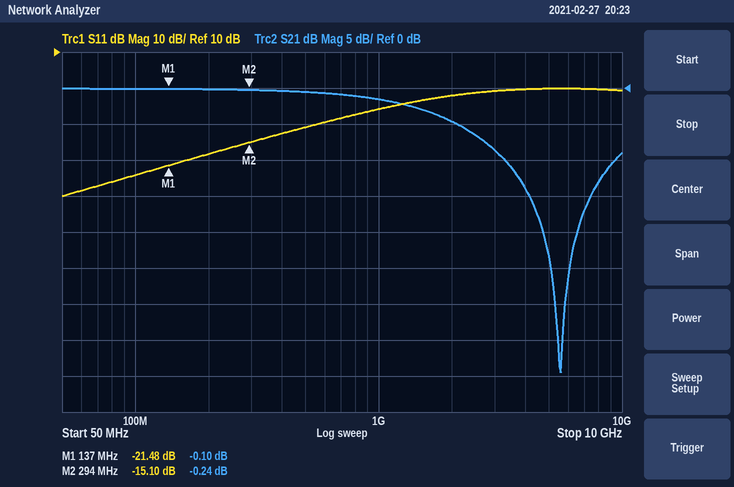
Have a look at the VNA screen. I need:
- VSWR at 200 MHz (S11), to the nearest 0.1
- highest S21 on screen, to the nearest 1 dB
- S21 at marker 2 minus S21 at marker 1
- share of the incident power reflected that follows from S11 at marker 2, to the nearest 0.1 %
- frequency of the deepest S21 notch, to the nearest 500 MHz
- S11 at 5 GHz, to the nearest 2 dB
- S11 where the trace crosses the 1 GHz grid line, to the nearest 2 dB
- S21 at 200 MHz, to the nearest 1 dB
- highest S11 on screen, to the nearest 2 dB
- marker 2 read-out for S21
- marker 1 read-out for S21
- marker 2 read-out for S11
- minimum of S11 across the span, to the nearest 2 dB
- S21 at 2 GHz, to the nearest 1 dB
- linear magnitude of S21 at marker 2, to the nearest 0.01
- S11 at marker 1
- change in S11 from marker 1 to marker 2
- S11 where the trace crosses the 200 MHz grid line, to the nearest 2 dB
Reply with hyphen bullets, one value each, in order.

- 1.3
- 0 dB
- -0.14 dB
- 3.1 %
- 5.5 GHz
- 0 dB
- -6 dB
- 0 dB
- 0 dB
- -0.24 dB
- -0.10 dB
- -15.10 dB
- -30 dB
- -5 dB
- 0.97
- -21.48 dB
- 6.38 dB
- -18 dB
